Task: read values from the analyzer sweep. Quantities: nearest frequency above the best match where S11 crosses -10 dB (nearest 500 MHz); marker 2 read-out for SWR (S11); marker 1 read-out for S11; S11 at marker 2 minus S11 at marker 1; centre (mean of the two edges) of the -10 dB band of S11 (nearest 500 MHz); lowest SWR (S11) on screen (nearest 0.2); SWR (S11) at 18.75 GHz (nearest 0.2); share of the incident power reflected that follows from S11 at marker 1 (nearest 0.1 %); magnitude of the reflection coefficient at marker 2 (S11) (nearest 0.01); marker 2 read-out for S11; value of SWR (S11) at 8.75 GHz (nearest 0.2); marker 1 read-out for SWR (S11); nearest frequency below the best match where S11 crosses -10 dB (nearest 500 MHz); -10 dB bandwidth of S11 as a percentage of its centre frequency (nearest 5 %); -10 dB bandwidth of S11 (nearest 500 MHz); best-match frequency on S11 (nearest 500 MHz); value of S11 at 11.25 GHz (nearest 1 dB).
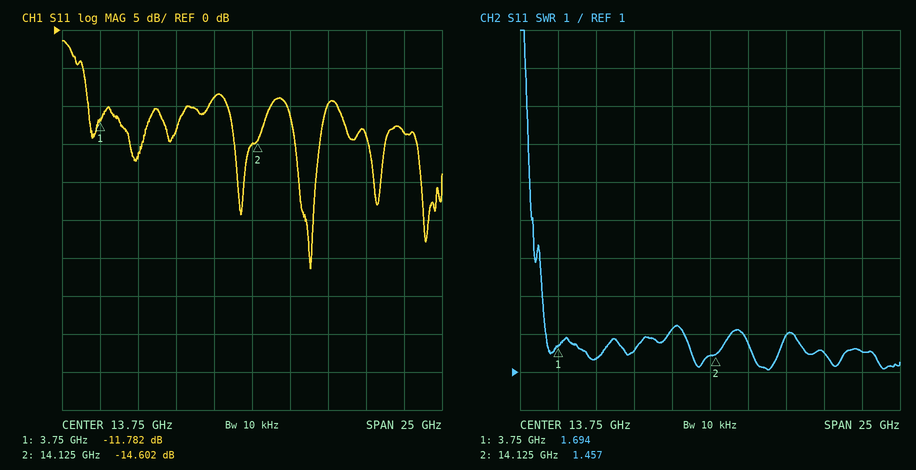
18.5 GHz
1.457
-11.782 dB
-2.820 dB
17.5 GHz
1.0
2.0
6.6 %
0.19
-14.602 dB
1.6
1.694
16.0 GHz
15 %
2.5 GHz
17.5 GHz
-9 dB
